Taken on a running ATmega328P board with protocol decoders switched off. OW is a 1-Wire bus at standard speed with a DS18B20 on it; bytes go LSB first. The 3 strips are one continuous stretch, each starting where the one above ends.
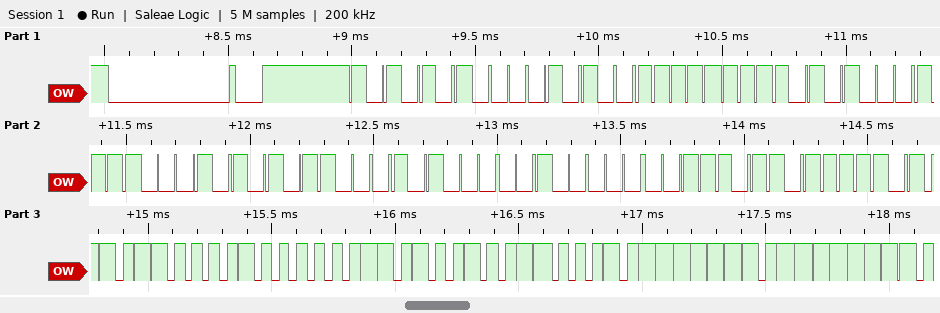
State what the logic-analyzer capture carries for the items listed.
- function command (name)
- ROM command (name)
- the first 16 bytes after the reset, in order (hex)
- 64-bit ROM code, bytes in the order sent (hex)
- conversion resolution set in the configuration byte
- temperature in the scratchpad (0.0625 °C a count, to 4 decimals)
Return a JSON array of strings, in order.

["Read Scratchpad", "Match ROM", "55 28 FF 15 8F 6A 14 04 DC BE 1A 02 4B 46 7F FF", "28 FF 15 8F 6A 14 04 DC", "12 bits", "33.6250 °C"]
